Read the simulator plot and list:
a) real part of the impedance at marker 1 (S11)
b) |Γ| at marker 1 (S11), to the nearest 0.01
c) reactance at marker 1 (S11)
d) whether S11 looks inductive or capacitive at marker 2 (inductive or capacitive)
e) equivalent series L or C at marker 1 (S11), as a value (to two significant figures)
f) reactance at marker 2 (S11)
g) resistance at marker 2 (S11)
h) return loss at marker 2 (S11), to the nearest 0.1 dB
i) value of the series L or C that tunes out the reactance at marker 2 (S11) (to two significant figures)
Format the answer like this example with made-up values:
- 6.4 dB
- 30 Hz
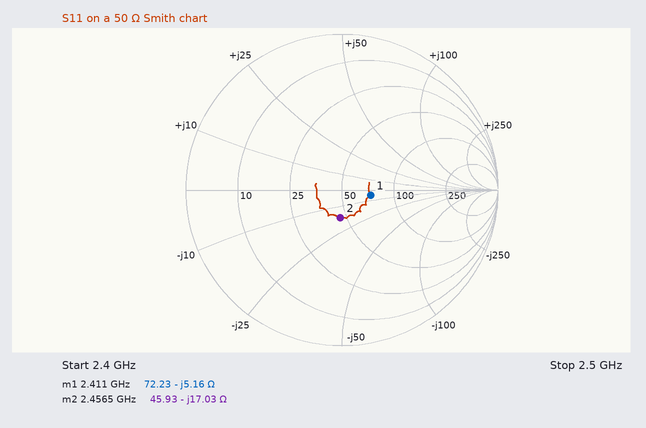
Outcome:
- 72.23 Ω
- 0.19
- -5.16 Ω
- capacitive
- 13 pF
- -17.03 Ω
- 45.93 Ω
- 14.9 dB
- 1.1 nH
